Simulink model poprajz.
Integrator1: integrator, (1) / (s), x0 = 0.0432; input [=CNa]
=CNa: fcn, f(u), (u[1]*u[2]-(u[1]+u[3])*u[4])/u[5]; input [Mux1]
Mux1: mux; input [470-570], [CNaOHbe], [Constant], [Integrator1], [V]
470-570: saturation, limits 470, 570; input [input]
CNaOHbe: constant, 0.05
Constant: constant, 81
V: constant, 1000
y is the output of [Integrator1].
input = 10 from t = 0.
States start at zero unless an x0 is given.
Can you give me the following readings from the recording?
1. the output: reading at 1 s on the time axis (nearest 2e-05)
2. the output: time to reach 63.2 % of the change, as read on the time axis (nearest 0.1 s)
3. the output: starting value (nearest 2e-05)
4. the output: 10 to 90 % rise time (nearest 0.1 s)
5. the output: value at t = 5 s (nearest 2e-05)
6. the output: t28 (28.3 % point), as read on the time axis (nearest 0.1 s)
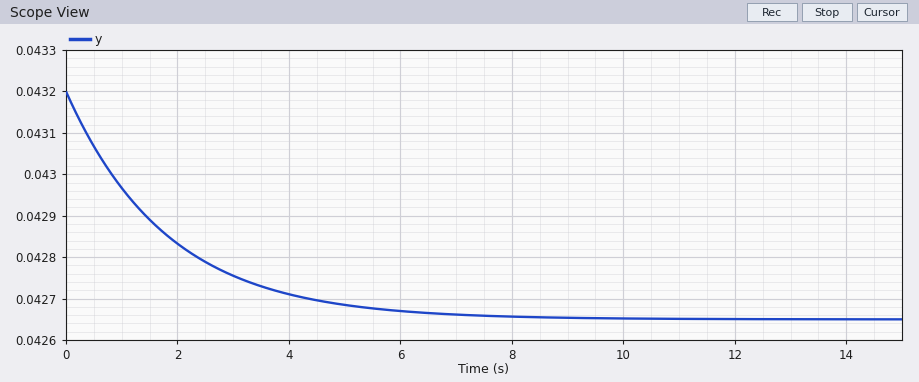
0.04296
1.8 s
0.04320
4.0 s
0.04268
0.6 s
